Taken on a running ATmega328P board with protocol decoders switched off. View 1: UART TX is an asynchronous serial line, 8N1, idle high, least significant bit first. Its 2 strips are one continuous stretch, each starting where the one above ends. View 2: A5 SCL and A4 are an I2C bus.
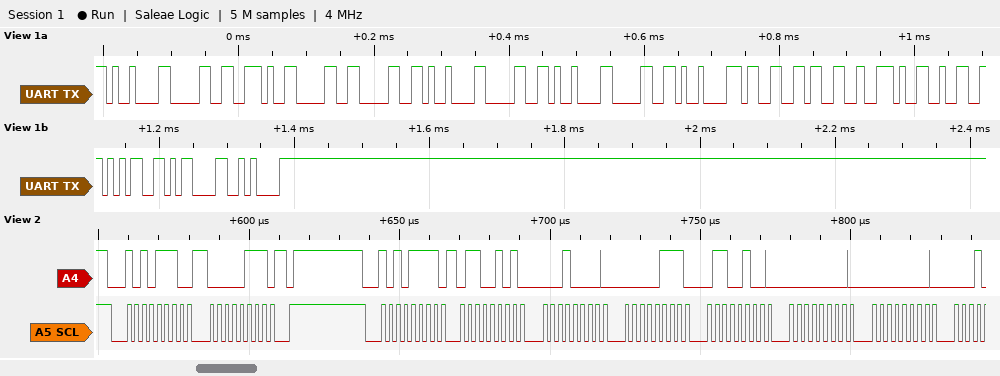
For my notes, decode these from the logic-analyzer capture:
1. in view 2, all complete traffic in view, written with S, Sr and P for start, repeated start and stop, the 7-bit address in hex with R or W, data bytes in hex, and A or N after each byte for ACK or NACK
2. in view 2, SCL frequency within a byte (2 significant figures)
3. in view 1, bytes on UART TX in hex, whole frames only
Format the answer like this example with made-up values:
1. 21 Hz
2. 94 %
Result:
1. S 57W A 07 A P S 57R A 65 A 10 A 07 A 64 A 00 A 00 A
2. 400 kHz
3. 09 30 2E 30 30 09 30 09 30 09 33 33 2E 32 35 0D 0A
